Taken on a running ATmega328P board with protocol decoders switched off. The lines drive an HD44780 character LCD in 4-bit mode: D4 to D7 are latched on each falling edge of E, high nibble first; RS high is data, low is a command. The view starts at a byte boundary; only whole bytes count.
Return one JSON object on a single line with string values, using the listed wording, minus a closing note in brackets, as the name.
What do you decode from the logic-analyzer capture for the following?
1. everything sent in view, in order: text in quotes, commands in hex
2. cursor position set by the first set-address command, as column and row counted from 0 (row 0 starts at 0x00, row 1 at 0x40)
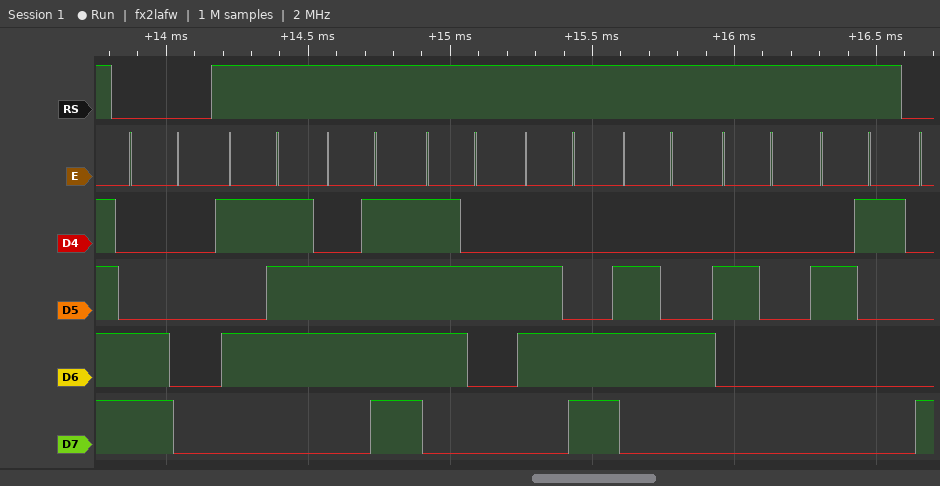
{"everything sent in view, in order: text in quotes, commands in hex": "0xC0 \"World !\"", "cursor position set by the first set-address command, as column and row counted from 0": "column 0, row 1"}
